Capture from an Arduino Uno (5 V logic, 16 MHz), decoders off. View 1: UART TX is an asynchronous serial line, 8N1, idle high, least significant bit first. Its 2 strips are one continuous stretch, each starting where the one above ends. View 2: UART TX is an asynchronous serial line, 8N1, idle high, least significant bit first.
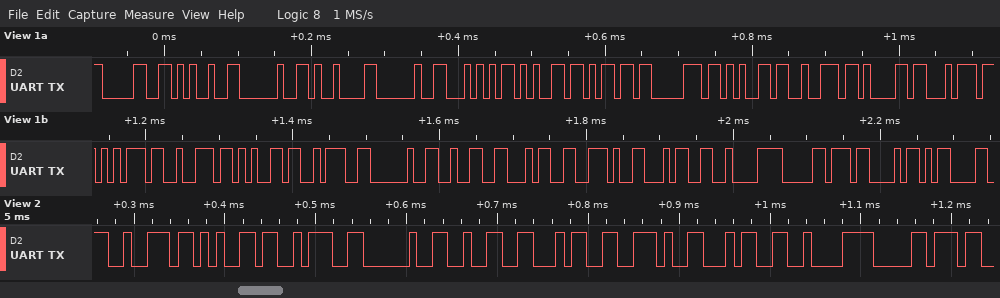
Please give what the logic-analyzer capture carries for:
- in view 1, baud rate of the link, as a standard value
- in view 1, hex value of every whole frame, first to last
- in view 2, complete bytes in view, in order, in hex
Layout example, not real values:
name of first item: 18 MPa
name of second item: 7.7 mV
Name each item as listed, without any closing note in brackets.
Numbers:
in view 1, baud rate of the link, as a standard value: 115200 baud
in view 1, hex value of every whole frame, first to last: 0x30 0x25 0x20 0x09 0x20 0x54 0x65 0x6D 0x70 0x65 0x72 0x61 0x74 0x75 0x72 0x65 0x3A 0x20 0x32 0x34 0x2E 0x34 0xC2 0xB0 0x43 0x0D
in view 2, complete bytes in view, in order, in hex: 72 65 3A 20 32 34 2E 34 C2 B0
